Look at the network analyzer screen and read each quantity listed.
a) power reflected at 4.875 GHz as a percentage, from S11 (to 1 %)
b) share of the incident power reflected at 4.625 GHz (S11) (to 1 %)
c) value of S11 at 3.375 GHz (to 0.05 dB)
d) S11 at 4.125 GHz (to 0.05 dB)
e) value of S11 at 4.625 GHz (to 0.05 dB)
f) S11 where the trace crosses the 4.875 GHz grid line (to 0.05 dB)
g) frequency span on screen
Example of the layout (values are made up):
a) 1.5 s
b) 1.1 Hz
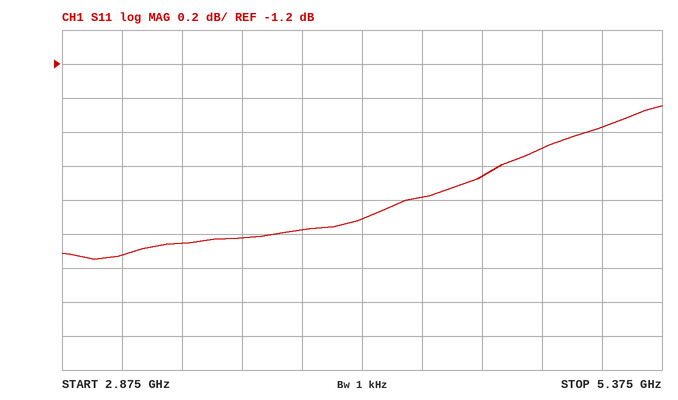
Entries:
a) 68 %
b) 65 %
c) -2.25 dB
d) -2.10 dB
e) -1.85 dB
f) -1.70 dB
g) 2.5 GHz
